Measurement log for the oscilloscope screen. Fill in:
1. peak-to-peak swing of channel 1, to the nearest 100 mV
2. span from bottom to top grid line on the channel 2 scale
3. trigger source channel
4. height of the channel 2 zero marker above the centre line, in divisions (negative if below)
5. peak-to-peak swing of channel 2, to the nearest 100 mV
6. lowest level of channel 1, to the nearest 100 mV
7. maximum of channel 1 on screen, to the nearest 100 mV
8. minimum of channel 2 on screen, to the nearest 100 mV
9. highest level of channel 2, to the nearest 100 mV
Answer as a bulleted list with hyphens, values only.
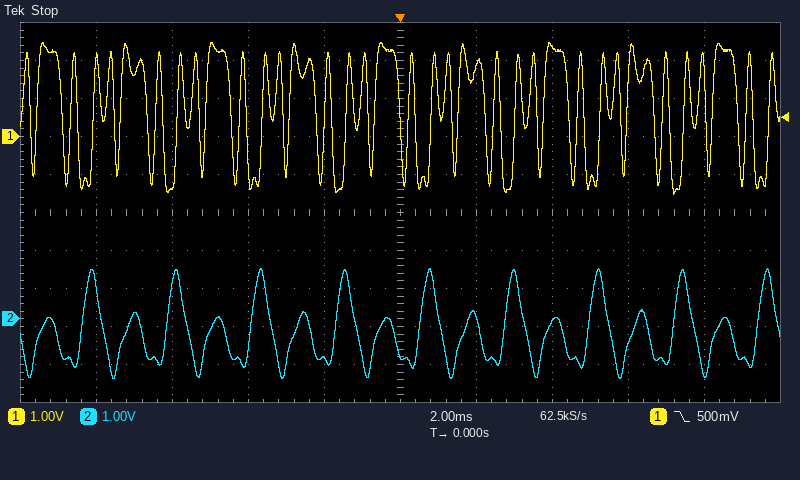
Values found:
- 4.0 V
- 10 V
- channel 1
- -2.8 div
- 2.9 V
- -1.5 V
- 2.5 V
- -1.6 V
- 1.3 V
